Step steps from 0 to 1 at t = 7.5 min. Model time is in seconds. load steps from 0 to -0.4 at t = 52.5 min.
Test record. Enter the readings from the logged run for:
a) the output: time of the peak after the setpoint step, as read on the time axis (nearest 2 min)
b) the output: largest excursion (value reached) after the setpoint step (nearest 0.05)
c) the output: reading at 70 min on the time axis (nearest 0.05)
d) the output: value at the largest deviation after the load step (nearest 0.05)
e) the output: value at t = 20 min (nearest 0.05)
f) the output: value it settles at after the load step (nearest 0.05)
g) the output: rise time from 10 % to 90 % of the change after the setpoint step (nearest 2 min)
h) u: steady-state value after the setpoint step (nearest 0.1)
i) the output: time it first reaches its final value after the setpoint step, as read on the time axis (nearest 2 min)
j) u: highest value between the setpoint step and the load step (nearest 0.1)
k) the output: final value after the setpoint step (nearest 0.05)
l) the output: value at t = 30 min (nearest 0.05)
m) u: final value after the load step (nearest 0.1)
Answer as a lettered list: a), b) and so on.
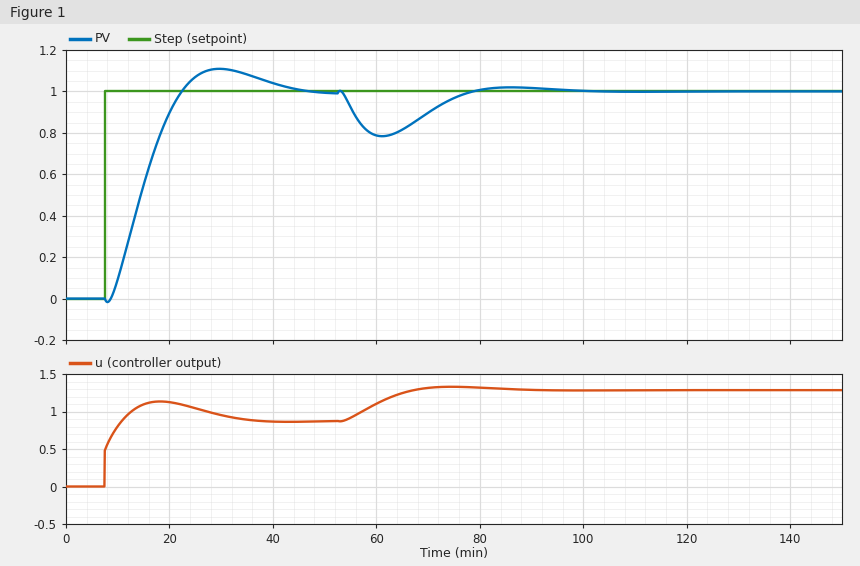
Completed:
a) 30 min
b) 1.10
c) 0.90
d) 0.80
e) 0.90
f) 1.00
g) 10 min
h) 0.9
i) 22 min
j) 1.1
k) 1.00
l) 1.10
m) 1.3
